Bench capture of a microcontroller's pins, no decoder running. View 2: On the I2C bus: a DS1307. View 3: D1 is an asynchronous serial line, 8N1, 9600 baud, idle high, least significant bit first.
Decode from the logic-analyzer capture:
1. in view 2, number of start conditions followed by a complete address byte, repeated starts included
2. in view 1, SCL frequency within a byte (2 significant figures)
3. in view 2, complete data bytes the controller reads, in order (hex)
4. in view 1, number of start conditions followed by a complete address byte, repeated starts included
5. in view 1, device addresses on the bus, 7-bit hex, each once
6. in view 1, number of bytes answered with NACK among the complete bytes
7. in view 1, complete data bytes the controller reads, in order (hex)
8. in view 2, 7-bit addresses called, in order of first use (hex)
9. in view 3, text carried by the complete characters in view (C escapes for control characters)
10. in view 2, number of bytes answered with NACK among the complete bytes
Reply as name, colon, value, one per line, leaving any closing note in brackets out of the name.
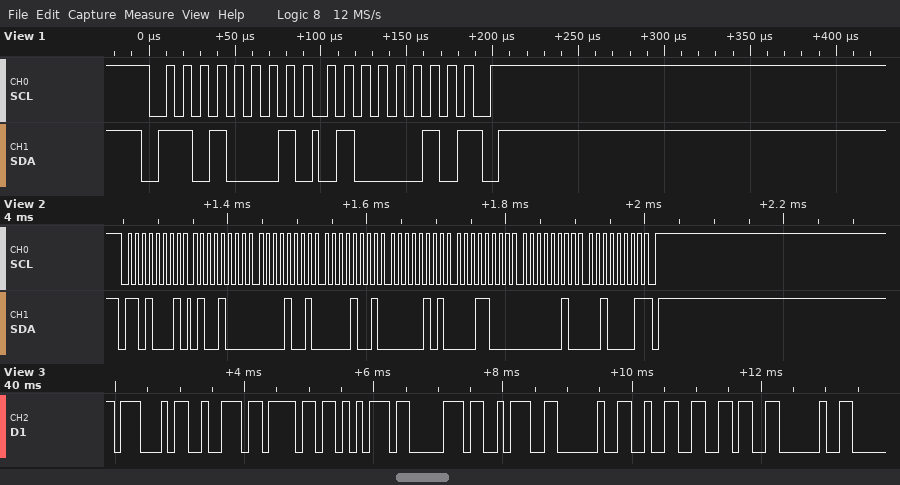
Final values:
in view 2, number of start conditions followed by a complete address byte, repeated starts included: 1
in view 1, SCL frequency within a byte: 100 kHz
in view 2, complete data bytes the controller reads, in order: 48 09 09 05 18 02 21
in view 1, number of start conditions followed by a complete address byte, repeated starts included: 1
in view 1, device addresses on the bus, 7-bit hex, each once: 0x68
in view 1, number of bytes answered with NACK among the complete bytes: 1
in view 1, complete data bytes the controller reads, in order: 42
in view 2, 7-bit addresses called, in order of first use: 0x68
in view 3, text carried by the complete characters in view: "Group: 26 "
in view 2, number of bytes answered with NACK among the complete bytes: 1
